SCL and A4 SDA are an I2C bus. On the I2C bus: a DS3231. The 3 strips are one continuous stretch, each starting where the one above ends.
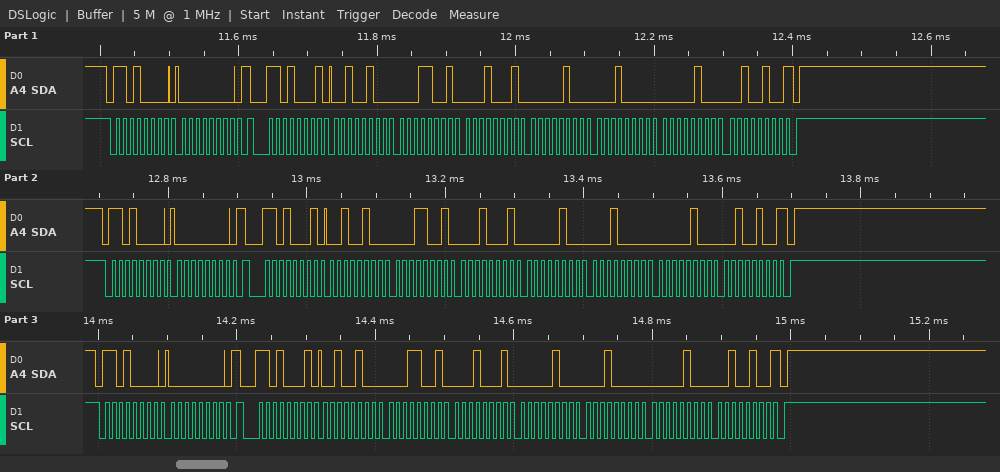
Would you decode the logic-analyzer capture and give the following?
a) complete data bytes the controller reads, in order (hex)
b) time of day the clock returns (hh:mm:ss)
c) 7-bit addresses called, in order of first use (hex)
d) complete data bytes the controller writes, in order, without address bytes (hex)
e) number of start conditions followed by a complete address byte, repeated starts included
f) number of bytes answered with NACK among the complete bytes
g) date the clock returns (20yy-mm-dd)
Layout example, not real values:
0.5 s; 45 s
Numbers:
24 19 11 04 10 04 24 24 19 11 04 10 04 24 24 19 11 04 10 04 24; 11:19:24; 0x68; 00 00 00; 6; 3; 2024-04-10
